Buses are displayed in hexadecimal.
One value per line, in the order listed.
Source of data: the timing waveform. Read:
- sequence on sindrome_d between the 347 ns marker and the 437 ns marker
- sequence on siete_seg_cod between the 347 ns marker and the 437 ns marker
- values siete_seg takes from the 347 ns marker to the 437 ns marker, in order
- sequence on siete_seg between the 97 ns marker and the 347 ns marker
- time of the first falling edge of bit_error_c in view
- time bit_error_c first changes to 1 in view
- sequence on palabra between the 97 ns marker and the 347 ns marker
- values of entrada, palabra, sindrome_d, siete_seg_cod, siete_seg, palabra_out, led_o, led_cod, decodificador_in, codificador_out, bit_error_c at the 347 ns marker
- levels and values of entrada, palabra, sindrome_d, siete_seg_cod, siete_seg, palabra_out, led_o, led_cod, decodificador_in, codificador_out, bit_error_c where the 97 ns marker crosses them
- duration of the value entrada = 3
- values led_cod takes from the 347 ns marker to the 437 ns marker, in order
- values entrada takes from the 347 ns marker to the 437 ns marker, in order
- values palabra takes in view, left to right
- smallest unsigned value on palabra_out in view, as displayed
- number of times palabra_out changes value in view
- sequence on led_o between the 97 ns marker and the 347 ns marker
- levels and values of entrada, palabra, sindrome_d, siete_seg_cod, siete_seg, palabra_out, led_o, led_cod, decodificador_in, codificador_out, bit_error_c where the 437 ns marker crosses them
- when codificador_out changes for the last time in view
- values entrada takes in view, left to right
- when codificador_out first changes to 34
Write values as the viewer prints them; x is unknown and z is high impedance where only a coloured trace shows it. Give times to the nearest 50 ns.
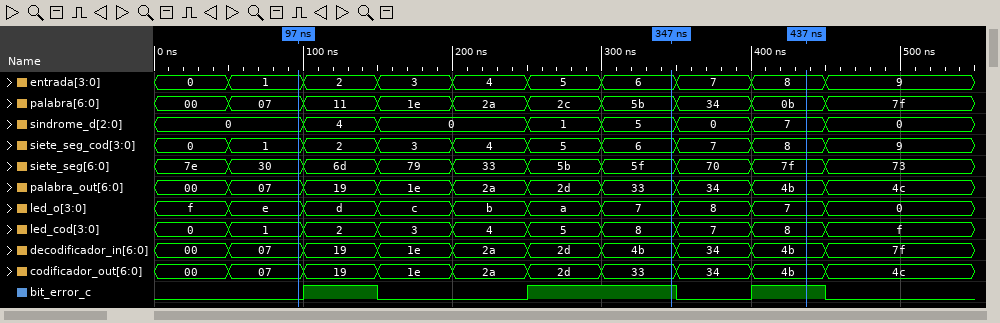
5, 0, 7
6, 7, 8
5f, 70, 7f
30, 6d, 79, 33, 5b, 5f
150 ns
100 ns
07, 11, 1e, 2a, 2c, 5b
entrada=6, palabra=5b, sindrome_d=5, siete_seg_cod=6, siete_seg=5f, palabra_out=33, led_o=7, led_cod=8, decodificador_in=4b, codificador_out=33, bit_error_c=1
entrada=1, palabra=07, sindrome_d=0, siete_seg_cod=1, siete_seg=30, palabra_out=07, led_o=e, led_cod=1, decodificador_in=07, codificador_out=07, bit_error_c=0
50 ns
8, 7, 8
6, 7, 8
00, 07, 11, 1e, 2a, 2c, 5b, 34, 0b, 7f
00
9
e, d, c, b, a, 7
entrada=8, palabra=0b, sindrome_d=7, siete_seg_cod=8, siete_seg=7f, palabra_out=4b, led_o=7, led_cod=8, decodificador_in=4b, codificador_out=4b, bit_error_c=1
450 ns
0, 1, 2, 3, 4, 5, 6, 7, 8, 9
350 ns
